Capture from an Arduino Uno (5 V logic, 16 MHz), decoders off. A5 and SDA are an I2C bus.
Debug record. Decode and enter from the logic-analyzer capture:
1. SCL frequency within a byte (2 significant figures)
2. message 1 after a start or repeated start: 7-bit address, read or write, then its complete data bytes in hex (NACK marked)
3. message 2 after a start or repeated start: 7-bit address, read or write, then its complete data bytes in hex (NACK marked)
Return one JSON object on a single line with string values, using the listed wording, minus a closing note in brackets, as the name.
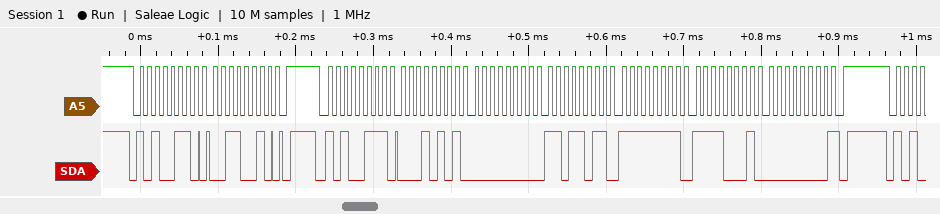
{"SCL frequency within a byte": "100 kHz", "message 1 after a start or repeated start: 7-bit address, read or write, then its complete data bytes in hex": "0x53 write: 32", "message 2 after a start or repeated start: 7-bit address, read or write, then its complete data bytes in hex": "0x53 read: 15 00 DB FF F1 00 NACK"}
